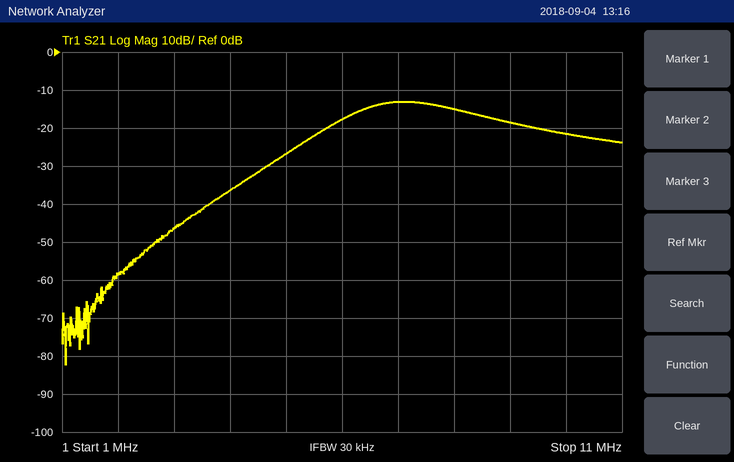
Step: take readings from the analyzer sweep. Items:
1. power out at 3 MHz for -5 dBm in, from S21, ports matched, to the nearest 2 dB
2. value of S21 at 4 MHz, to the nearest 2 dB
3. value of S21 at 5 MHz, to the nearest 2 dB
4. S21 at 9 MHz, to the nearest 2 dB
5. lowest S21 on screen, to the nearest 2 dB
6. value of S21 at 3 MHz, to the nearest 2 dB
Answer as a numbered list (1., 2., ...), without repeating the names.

1. -52 dBm
2. -36 dB
3. -26 dB
4. -18 dB
5. -82 dB
6. -46 dB
